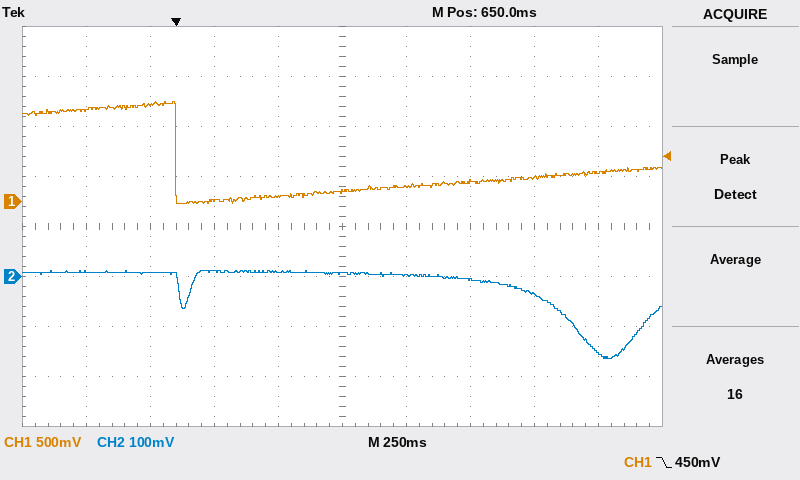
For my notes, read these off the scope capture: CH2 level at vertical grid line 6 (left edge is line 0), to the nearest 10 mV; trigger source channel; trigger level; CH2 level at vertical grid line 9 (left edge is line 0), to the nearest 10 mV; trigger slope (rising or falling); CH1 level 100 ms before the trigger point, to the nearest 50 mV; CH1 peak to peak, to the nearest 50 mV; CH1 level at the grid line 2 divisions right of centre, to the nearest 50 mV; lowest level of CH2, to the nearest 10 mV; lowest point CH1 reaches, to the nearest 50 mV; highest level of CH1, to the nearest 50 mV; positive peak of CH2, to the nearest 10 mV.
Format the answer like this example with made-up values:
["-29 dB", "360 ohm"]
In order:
["0 mV", "CH1", "450 mV", "-150 mV", "falling", "950 mV", "1.00 V", "200 mV", "-160 mV", "0 mV", "1.00 V", "10 mV"]
